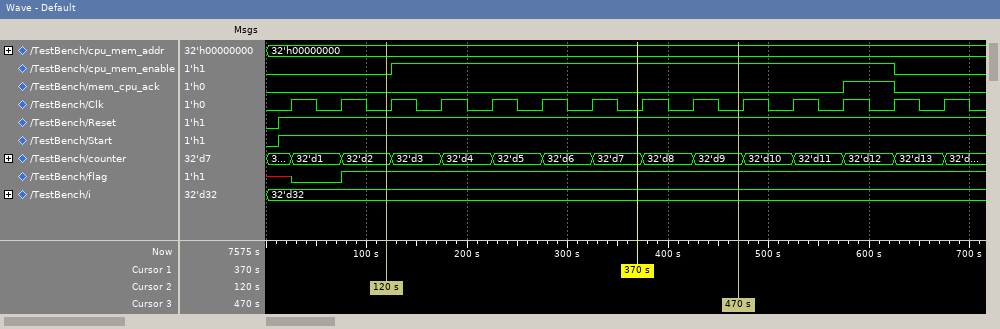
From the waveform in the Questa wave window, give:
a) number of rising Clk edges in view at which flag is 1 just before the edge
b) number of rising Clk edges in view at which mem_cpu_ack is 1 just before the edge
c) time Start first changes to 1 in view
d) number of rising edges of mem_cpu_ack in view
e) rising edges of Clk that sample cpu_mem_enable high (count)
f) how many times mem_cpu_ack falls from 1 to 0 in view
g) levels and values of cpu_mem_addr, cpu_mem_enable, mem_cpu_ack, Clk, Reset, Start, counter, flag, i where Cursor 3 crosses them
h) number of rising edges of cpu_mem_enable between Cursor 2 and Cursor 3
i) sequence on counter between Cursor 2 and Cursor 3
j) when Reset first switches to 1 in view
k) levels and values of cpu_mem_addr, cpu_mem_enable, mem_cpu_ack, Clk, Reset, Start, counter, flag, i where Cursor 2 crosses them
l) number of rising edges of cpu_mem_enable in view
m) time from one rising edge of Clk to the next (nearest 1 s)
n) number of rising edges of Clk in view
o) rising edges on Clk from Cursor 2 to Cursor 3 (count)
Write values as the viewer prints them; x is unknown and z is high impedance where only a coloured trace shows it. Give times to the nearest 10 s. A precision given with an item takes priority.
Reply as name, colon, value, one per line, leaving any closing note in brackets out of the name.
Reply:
number of rising Clk edges in view at which flag is 1 just before the edge: 12
number of rising Clk edges in view at which mem_cpu_ack is 1 just before the edge: 1
time Start first changes to 1 in view: 10 s
number of rising edges of mem_cpu_ack in view: 1
rising edges of Clk that sample cpu_mem_enable high: 10
how many times mem_cpu_ack falls from 1 to 0 in view: 1
levels and values of cpu_mem_addr, cpu_mem_enable, mem_cpu_ack, Clk, Reset, Start, counter, flag, i where Cursor 3 crosses them: cpu_mem_addr=32'h00000000, cpu_mem_enable=1, mem_cpu_ack=0, Clk=0, Reset=1, Start=1, counter=32'd9, flag=1, i=32'd32
number of rising edges of cpu_mem_enable between Cursor 2 and Cursor 3: 1
sequence on counter between Cursor 2 and Cursor 3: 32'd2, 32'd3, 32'd4, 32'd5, 32'd6, 32'd7, 32'd8, 32'd9
when Reset first switches to 1 in view: 10 s
levels and values of cpu_mem_addr, cpu_mem_enable, mem_cpu_ack, Clk, Reset, Start, counter, flag, i where Cursor 2 crosses them: cpu_mem_addr=32'h00000000, cpu_mem_enable=0, mem_cpu_ack=0, Clk=0, Reset=1, Start=1, counter=32'd2, flag=1, i=32'd32
number of rising edges of cpu_mem_enable in view: 1
time from one rising edge of Clk to the next: 50 s
number of rising edges of Clk in view: 14
rising edges on Clk from Cursor 2 to Cursor 3: 7
